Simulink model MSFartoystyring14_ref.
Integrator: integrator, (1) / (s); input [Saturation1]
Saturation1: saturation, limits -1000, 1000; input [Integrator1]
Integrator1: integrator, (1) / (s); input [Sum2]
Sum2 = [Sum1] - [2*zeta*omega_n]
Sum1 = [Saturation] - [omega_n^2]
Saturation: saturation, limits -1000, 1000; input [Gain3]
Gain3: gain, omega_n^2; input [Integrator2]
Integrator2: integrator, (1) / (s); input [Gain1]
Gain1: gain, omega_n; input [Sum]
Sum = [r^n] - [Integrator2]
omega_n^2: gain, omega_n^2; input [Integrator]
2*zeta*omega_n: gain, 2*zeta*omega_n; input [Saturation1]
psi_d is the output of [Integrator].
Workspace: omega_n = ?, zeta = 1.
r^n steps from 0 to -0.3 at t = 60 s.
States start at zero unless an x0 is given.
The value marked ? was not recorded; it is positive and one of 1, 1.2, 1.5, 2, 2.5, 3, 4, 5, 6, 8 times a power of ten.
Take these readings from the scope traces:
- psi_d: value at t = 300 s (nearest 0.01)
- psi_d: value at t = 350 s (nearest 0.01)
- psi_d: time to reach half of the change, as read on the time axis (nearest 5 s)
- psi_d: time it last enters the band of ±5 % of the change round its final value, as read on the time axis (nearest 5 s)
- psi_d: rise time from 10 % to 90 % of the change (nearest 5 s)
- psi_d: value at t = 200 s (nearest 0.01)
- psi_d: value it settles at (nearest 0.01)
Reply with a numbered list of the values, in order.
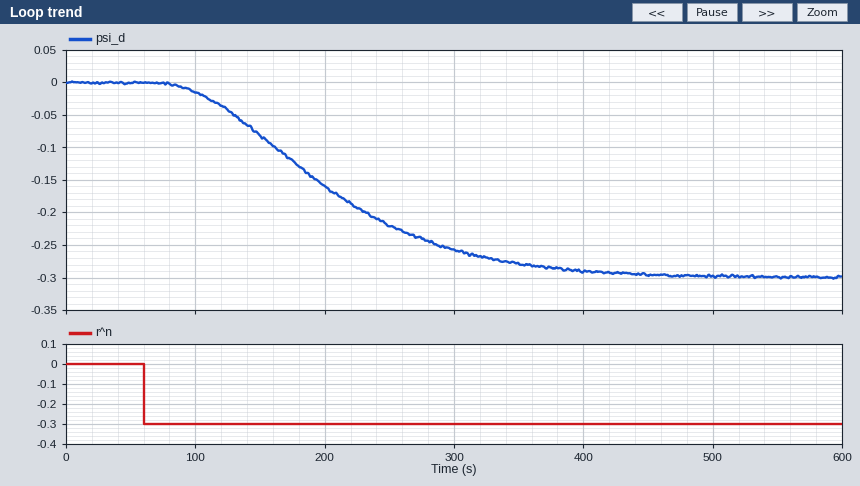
1. -0.26
2. -0.28
3. 195 s
4. 375 s
5. 210 s
6. -0.16
7. -0.30
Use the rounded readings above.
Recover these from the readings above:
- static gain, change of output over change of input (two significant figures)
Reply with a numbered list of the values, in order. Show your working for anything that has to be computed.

1. (-0.3 - 0) / (-0.3 - 0) = 1.0
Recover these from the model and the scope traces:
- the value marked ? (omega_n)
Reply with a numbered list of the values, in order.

1. 0.02
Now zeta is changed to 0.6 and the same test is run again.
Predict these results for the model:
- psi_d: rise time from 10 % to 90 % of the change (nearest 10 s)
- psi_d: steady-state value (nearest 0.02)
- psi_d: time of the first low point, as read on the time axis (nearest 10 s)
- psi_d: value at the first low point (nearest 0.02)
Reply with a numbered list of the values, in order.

1. 130 s
2. -0.30
3. 330 s
4. -0.32
